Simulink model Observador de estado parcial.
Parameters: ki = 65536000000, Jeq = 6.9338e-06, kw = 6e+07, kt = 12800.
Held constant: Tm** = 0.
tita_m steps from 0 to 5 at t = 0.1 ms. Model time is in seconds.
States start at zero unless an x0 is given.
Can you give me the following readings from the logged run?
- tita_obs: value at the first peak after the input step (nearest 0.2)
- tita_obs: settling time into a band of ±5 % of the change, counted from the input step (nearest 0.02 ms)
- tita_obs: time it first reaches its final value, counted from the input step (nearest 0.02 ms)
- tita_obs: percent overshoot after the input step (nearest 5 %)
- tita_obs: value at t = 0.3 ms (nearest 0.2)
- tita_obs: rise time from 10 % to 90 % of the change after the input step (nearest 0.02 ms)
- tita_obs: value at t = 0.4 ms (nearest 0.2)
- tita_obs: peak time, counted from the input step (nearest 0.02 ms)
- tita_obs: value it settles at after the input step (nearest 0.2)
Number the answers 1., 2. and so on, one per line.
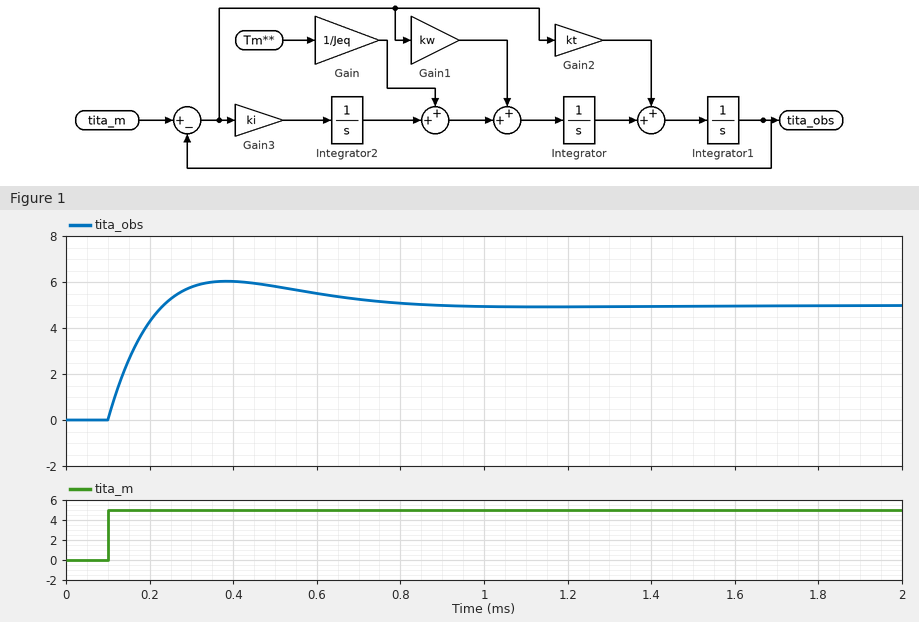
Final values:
1. 6.0
2. 0.60 ms
3. 0.14 ms
4. 20 %
5. 5.8
6. 0.10 ms
7. 6.0
8. 0.28 ms
9. 5.0
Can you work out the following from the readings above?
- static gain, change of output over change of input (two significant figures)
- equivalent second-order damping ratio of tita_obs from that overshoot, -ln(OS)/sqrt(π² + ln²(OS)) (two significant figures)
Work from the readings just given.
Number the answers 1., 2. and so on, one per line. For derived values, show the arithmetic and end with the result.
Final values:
1. (5 - 0) / (5 - 0) = 1.0
2. ln(0.2) = -1.609; 1.609 / sqrt(9.870 + 2.590) = 0.46
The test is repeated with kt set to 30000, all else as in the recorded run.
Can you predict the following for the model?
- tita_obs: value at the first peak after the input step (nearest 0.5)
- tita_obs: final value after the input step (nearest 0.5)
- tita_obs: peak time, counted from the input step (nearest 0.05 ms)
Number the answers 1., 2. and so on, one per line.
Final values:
1. 5.5
2. 5.0
3. 0.20 ms
